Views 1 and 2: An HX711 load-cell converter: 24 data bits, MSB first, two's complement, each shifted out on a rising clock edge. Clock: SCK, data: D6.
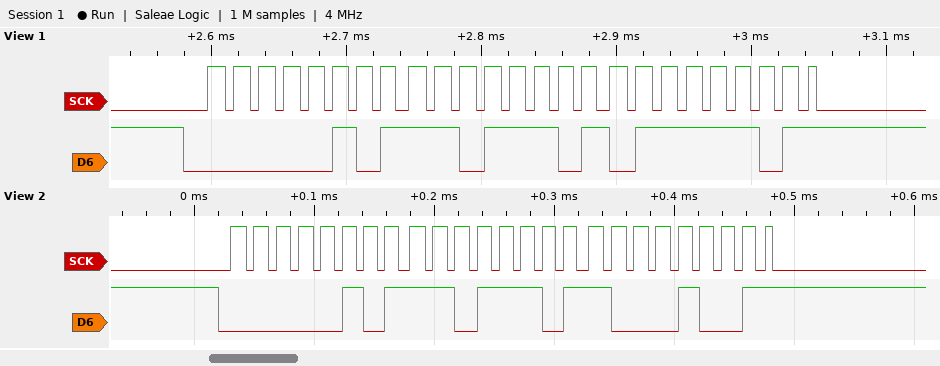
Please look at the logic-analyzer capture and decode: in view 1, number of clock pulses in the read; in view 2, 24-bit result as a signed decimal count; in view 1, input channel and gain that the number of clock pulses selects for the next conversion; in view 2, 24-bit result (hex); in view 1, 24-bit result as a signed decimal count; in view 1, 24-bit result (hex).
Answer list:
25
384393
channel A, gain 128
0x05DD89
384381
0x05DD7D
